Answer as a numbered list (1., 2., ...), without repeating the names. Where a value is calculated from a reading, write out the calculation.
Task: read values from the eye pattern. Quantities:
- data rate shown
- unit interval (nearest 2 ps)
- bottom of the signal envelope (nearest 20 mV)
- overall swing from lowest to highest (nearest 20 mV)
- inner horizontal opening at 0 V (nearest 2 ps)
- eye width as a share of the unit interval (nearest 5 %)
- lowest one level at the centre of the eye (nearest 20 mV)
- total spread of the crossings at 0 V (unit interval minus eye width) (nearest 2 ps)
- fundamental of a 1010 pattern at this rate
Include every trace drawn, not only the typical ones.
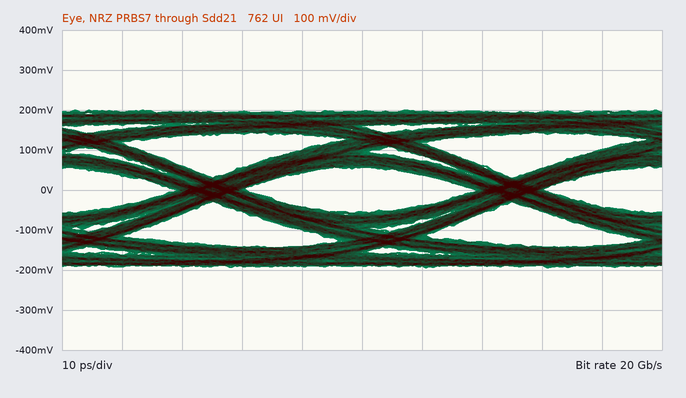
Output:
1. 20 Gb/s
2. 50 ps
3. -200 mV
4. 400 mV
5. 38 ps
6. 38 ps / 50 ps ≈ 76.0 %, so 75 % to the nearest 5 %
7. 60 mV
8. 12 ps
9. 10 GHz
